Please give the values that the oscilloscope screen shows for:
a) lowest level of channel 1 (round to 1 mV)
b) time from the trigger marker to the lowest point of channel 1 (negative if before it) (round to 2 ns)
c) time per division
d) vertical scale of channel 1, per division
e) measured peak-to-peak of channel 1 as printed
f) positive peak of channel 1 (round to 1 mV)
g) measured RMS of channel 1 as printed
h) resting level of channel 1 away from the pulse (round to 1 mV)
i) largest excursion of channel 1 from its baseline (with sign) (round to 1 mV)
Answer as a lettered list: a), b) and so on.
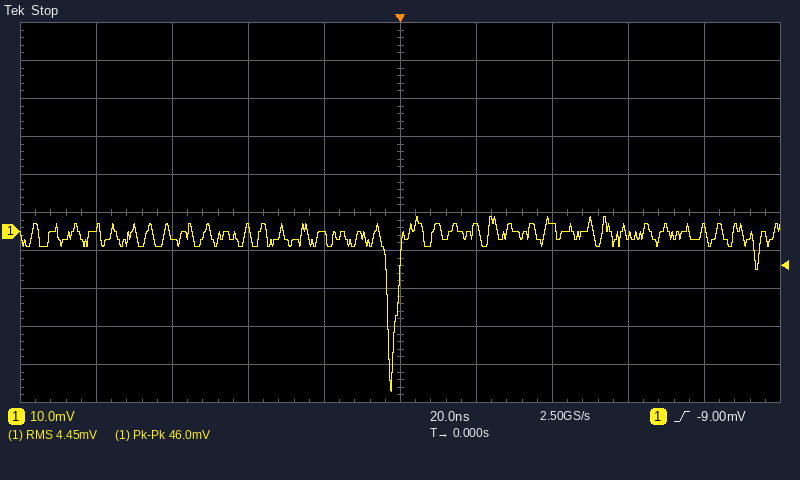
a) -42 mV
b) -2 ns
c) 20 ns
d) 10 mV
e) 46.0 mV
f) 4 mV
g) 4.45 mV
h) -1 mV
i) -41 mV
